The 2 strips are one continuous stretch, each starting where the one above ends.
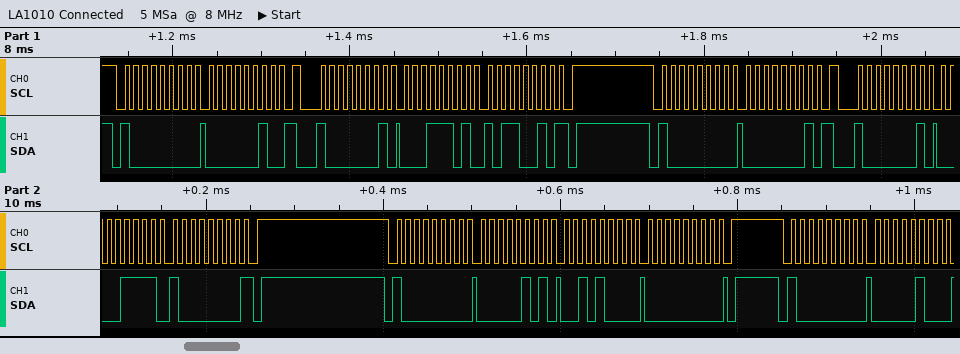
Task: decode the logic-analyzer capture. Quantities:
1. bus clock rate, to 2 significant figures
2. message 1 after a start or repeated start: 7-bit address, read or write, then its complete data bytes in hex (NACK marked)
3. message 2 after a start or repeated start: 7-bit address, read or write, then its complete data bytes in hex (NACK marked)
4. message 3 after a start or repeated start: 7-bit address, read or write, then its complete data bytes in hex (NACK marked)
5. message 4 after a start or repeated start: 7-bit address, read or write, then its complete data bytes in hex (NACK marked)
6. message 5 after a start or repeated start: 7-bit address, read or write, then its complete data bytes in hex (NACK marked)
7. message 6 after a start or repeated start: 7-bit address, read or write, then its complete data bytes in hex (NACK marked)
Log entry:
100 kHz
0x40 write: 02
0x40 read: 1D B2 NACK
0x40 write: 01
0x40 read: 0F 80 NACK
0x40 write: 05 28 00
0x40 write: 04
